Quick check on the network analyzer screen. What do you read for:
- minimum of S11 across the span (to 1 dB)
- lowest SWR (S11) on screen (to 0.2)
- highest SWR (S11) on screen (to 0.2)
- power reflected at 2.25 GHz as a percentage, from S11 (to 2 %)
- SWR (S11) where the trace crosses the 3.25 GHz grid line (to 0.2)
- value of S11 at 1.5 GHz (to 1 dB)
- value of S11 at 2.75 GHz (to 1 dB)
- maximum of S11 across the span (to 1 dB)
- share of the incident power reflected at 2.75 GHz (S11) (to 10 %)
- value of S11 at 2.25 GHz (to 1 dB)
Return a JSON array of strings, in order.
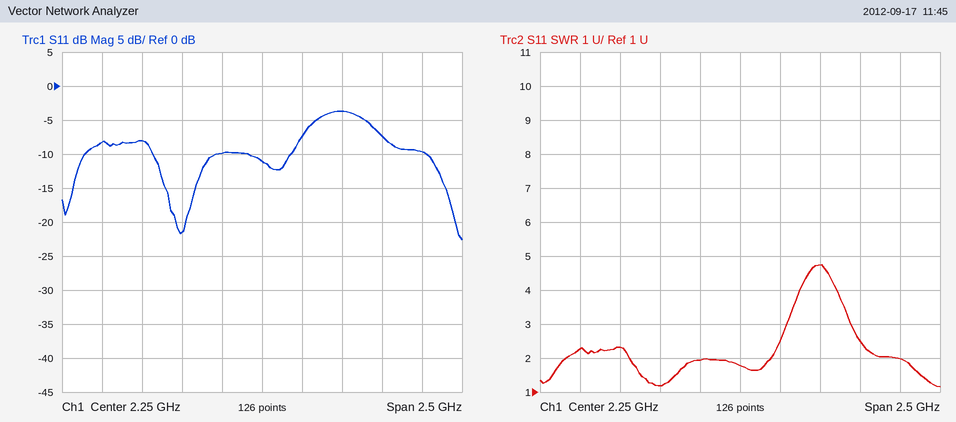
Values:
["-23 dB", "1.2", "4.8", "8 %", "2.0", "-8 dB", "-4 dB", "-4 dB", "40 %", "-11 dB"]
